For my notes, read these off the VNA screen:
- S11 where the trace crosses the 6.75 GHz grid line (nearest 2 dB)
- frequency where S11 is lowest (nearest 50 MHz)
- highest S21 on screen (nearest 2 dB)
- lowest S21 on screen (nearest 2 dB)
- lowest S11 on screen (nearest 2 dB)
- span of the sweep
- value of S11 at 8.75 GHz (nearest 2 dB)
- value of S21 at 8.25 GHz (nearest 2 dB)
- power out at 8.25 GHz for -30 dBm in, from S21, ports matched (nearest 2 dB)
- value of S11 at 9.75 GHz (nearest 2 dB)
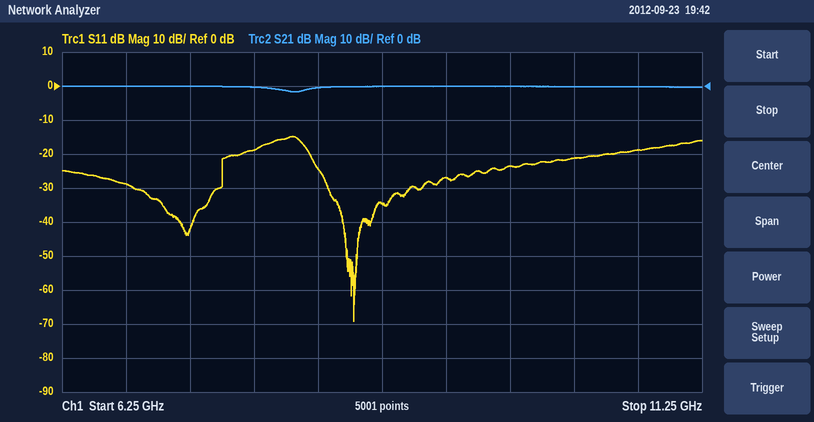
-28 dB
8.55 GHz
0 dB
-2 dB
-70 dB
5 GHz
-34 dB
0 dB
-30 dBm
-24 dB
